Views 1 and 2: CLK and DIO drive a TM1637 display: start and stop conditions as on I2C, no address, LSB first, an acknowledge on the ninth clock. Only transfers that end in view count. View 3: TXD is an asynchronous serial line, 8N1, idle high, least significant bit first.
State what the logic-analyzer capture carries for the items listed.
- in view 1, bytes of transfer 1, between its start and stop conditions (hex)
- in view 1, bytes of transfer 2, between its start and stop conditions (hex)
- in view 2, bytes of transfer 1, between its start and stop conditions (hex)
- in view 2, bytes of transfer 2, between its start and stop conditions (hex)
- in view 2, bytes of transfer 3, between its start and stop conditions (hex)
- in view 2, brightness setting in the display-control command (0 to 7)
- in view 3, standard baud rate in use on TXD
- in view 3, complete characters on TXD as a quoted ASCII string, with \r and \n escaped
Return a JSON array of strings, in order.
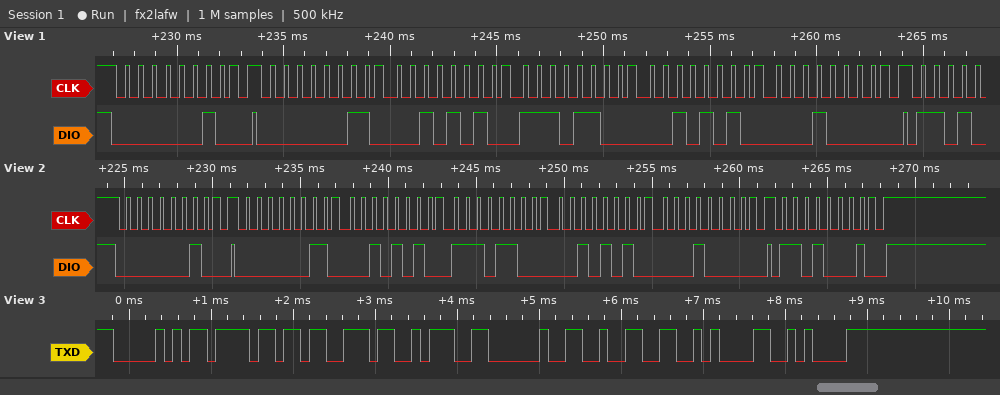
["40", "C0 54 37 54 08", "40", "C0 54 37 54 08", "8B", "3", "9600 baud", "\"Pos: 2\\n\\n\""]
